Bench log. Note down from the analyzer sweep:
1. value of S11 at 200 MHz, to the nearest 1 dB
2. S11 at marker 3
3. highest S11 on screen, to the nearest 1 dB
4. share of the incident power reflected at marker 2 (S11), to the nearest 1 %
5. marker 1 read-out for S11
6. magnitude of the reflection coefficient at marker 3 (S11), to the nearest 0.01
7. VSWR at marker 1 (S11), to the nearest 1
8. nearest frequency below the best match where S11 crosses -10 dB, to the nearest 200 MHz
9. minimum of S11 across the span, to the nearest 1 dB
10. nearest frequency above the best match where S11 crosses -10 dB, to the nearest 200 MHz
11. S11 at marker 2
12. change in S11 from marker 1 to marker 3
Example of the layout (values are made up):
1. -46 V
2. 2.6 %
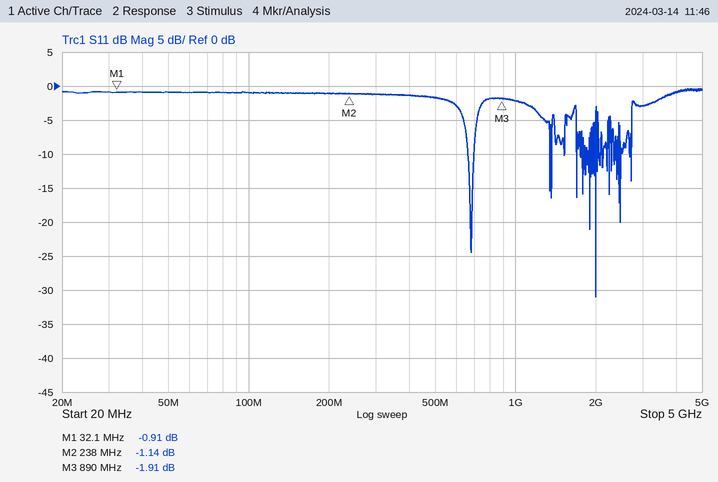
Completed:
1. -1 dB
2. -1.91 dB
3. 0 dB
4. 77 %
5. -0.91 dB
6. 0.80
7. 19
8. 2.0 GHz
9. -31 dB
10. 2.0 GHz
11. -1.14 dB
12. -1.00 dB
